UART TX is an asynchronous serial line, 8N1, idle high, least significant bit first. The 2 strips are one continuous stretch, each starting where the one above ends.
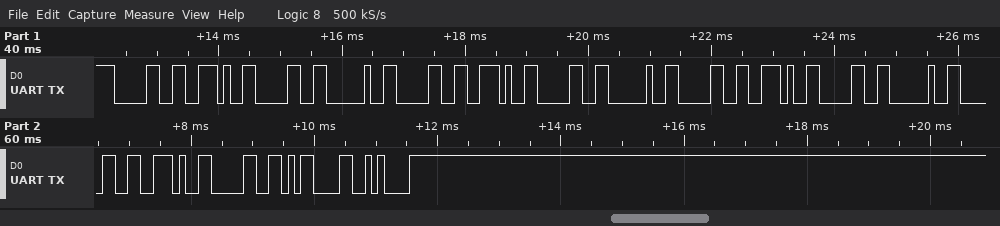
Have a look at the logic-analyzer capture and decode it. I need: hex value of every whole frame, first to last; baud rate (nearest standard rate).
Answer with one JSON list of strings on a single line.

["0x30 0x2E 0x30 0x20 0x30 0x2E 0x30 0x20 0x30 0x2E 0x30 0x20 0x30 0x2E 0x30 0x0D 0x0A", "9600 baud"]
